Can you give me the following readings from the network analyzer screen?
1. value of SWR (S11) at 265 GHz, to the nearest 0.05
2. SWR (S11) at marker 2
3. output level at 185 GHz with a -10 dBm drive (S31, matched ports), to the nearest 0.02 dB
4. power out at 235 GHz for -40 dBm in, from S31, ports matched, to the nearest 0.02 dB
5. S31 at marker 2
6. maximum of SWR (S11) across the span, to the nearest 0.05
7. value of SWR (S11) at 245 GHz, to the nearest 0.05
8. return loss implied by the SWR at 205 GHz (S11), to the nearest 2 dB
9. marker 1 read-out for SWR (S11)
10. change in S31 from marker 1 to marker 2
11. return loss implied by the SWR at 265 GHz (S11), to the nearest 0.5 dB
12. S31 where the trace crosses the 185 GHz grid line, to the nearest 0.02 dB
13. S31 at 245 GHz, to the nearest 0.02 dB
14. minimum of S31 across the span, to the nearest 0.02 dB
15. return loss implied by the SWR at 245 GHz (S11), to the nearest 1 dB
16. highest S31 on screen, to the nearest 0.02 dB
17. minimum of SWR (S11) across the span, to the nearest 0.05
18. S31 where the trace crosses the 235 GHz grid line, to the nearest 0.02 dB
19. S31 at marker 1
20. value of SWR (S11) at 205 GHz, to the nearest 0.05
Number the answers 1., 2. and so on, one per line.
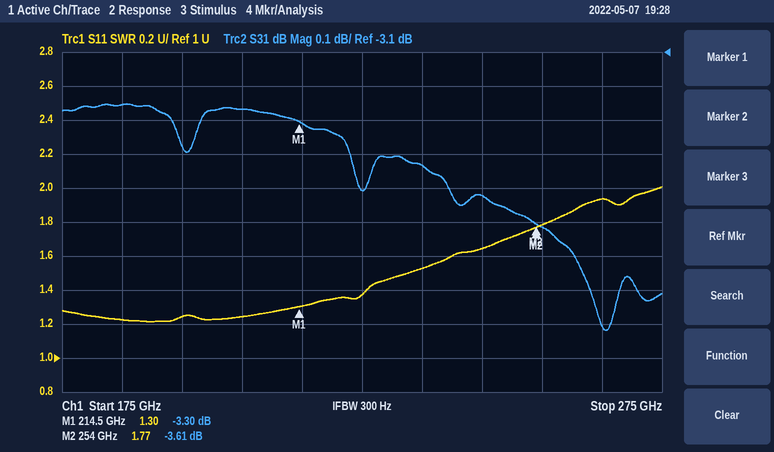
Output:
1. 1.95
2. 1.77
3. -13.26 dBm
4. -43.44 dBm
5. -3.61 dB
6. 2.00
7. 1.65
8. 20 dB
9. 1.30
10. -0.31 dB
11. 10.0 dB
12. -3.26 dB
13. -3.52 dB
14. -3.92 dB
15. 12 dB
16. -3.26 dB
17. 1.20
18. -3.44 dB
19. -3.30 dB
20. 1.25
